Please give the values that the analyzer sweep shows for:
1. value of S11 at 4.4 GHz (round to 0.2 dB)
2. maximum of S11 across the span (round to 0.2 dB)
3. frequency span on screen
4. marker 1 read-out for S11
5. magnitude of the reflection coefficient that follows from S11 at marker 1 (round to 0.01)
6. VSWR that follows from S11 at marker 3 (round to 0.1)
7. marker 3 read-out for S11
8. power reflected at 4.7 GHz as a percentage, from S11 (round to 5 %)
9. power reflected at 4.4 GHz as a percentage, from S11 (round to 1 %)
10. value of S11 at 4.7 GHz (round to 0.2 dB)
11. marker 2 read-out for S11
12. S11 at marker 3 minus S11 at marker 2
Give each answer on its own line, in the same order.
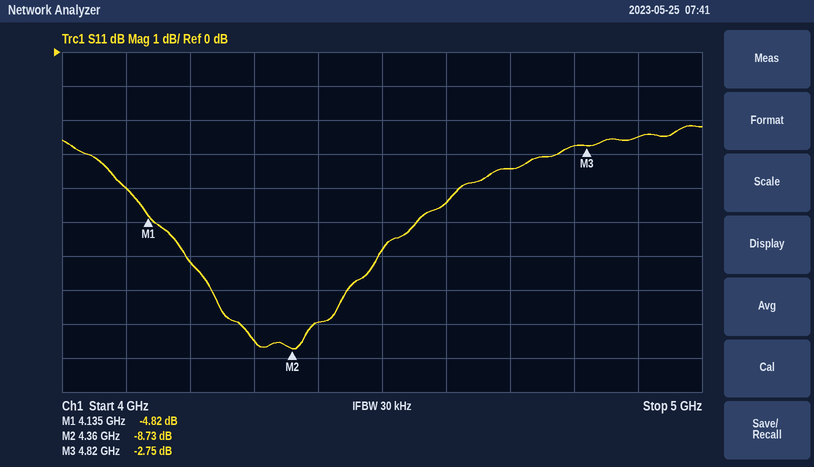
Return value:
-8.0 dB
-2.2 dB
1 GHz
-4.82 dB
0.57
6.4
-2.75 dB
45 %
16 %
-3.4 dB
-8.73 dB
5.98 dB
